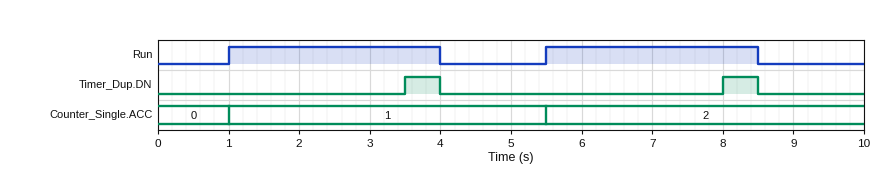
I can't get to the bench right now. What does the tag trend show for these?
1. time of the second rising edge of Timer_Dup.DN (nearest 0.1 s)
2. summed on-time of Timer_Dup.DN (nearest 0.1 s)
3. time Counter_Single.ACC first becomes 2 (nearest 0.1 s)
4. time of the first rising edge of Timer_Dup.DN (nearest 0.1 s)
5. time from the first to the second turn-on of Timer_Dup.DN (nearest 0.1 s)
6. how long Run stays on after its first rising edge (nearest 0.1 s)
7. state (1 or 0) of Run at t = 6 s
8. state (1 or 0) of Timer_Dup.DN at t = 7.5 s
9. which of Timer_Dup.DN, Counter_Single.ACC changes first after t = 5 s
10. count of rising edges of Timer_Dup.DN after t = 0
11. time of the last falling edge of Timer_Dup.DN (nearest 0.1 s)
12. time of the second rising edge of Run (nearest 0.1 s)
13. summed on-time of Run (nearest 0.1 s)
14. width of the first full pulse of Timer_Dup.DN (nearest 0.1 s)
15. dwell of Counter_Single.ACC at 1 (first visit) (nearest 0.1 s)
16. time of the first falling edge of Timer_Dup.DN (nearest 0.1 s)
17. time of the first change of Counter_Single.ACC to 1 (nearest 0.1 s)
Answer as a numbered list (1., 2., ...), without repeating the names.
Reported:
1. 8.0 s
2. 1.0 s
3. 5.5 s
4. 3.5 s
5. 4.5 s
6. 3.0 s
7. 1
8. 0
9. Counter_Single.ACC
10. 2
11. 8.5 s
12. 5.5 s
13. 6.0 s
14. 0.5 s
15. 4.5 s
16. 4.0 s
17. 1.0 s
